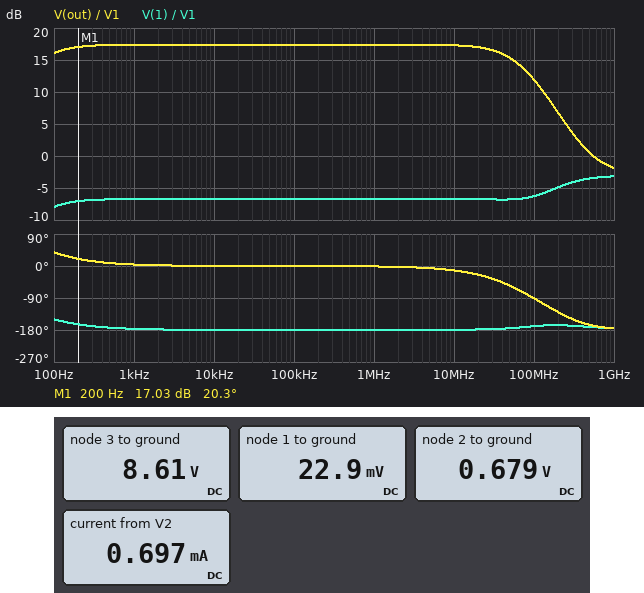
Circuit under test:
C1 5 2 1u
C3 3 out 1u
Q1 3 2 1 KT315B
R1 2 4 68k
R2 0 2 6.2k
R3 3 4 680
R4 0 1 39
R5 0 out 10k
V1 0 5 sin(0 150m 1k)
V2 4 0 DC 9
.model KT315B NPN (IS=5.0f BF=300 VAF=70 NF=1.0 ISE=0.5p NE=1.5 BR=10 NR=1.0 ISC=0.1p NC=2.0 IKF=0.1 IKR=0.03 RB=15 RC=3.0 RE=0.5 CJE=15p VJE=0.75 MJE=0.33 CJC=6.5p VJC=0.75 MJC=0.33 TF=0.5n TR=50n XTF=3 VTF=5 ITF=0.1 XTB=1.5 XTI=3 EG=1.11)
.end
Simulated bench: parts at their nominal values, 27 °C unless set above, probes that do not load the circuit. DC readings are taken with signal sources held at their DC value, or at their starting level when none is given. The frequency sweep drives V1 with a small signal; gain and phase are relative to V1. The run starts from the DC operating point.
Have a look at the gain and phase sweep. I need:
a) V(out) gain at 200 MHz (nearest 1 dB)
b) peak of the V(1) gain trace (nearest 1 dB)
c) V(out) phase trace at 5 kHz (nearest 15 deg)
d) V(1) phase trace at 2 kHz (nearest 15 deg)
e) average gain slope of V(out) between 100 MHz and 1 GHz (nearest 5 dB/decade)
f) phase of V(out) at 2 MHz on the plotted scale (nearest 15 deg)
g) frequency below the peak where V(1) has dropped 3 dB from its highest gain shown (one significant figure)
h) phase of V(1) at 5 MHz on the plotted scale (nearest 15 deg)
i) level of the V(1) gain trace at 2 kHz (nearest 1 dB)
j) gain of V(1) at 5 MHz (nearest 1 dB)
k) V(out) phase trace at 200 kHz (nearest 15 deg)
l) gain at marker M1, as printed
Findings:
7 dB
-3 dB
0 deg
-180 deg
-15 dB/decade
0 deg
100 MHz
-180 deg
-7 dB
-7 dB
0 deg
17.03 dB
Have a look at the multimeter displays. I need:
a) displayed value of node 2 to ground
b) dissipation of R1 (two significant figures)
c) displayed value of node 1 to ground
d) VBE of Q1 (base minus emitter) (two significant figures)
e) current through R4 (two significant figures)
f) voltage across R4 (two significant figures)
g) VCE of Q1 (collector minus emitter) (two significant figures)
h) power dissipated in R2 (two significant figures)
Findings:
0.679 V
1.0 mW
22.9 mV
660 mV
590 µA
23 mV
8.6 V
74 µW
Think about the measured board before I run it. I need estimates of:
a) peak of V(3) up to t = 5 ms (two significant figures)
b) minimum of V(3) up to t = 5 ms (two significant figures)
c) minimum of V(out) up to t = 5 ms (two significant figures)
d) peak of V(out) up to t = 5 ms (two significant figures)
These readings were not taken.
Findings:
9.0 V
6.9 V
-1.7 V
460 mV
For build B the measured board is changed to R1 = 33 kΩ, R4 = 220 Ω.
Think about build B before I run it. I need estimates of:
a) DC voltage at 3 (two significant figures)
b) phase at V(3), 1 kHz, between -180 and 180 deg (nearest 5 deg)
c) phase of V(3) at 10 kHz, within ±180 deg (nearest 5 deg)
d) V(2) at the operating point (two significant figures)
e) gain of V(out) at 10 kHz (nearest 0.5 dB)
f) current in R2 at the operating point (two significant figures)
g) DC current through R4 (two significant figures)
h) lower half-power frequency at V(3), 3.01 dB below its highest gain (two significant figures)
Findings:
7.4 V
0 deg
0 deg
1.2 V
8.5 dB
200 µA
2.4 mA
38 Hz
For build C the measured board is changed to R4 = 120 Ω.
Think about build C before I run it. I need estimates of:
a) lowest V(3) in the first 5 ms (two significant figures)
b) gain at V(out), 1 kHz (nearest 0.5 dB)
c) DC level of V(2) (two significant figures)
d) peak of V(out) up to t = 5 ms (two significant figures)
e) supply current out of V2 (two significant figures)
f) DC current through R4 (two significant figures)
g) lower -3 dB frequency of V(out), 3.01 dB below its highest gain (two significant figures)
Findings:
8.1 V
10.5 dB
700 mV
280 mV
520 µA
410 µA
47 Hz
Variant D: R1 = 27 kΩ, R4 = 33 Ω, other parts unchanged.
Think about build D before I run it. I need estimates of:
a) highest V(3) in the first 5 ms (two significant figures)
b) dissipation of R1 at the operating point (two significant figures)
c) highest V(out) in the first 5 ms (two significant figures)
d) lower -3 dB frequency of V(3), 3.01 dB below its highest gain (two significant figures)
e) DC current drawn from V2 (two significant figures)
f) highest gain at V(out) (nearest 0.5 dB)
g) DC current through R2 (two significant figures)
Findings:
5.3 V
2.3 mW
3.0 V
78 Hz
10 mA
24.5 dB
170 µA
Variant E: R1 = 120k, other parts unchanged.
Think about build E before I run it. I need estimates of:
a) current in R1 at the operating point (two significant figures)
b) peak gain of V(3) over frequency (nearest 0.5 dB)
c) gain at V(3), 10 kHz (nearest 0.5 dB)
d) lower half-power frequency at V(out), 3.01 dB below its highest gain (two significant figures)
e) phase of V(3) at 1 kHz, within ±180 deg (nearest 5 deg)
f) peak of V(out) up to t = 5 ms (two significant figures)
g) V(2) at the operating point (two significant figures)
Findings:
71 µA
-2.5 dB
-49.0 dB
58 MHz
0 deg
2.0 mV
440 mV
